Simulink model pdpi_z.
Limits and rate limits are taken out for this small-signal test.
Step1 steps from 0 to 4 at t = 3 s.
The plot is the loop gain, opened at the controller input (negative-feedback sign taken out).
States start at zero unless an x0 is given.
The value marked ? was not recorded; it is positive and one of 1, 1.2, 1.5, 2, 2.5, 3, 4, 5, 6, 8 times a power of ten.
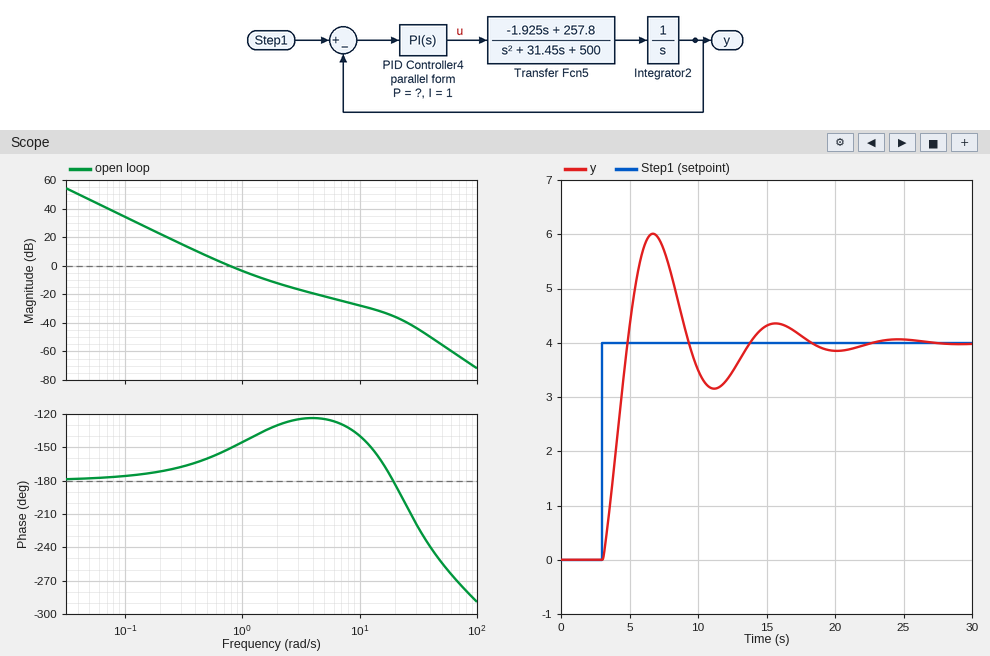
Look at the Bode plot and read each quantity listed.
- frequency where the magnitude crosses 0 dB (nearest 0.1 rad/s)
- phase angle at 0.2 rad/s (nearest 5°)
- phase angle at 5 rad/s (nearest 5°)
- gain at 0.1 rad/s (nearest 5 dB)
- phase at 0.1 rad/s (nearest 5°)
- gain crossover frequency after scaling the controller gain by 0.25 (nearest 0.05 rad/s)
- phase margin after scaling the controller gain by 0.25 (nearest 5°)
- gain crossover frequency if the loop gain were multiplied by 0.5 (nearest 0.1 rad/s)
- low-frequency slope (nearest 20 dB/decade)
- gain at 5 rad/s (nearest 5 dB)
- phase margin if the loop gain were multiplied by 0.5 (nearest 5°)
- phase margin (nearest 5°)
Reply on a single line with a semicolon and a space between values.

0.8 rad/s; -170°; -125°; 35 dB; -175°; 0.35 rad/s; 15°; 0.5 rad/s; -40 dB/decade; -20 dB; 20°; 30°
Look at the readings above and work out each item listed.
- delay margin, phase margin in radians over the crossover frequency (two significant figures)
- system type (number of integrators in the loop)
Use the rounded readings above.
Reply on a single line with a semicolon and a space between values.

0.65 s; 2
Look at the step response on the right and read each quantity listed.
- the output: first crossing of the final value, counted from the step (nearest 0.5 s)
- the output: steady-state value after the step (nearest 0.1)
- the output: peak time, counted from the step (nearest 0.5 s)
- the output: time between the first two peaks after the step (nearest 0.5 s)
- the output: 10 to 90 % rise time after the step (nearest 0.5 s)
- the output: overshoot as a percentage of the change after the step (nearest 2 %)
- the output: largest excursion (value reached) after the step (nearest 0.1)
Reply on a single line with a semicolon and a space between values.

2.0 s; 4.0; 3.5 s; 9.0 s; 1.5 s; 50 %; 6.0
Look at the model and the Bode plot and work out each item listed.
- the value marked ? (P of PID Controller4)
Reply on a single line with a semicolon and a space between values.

0.8
